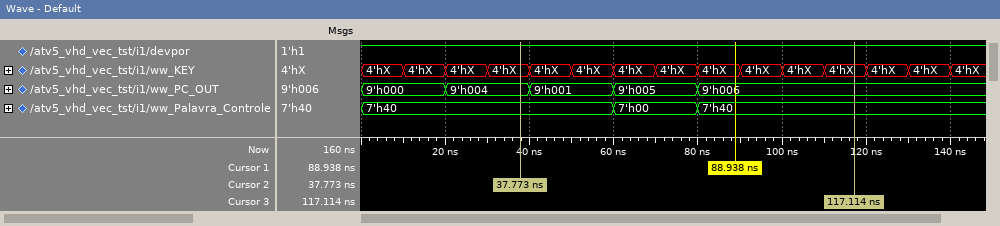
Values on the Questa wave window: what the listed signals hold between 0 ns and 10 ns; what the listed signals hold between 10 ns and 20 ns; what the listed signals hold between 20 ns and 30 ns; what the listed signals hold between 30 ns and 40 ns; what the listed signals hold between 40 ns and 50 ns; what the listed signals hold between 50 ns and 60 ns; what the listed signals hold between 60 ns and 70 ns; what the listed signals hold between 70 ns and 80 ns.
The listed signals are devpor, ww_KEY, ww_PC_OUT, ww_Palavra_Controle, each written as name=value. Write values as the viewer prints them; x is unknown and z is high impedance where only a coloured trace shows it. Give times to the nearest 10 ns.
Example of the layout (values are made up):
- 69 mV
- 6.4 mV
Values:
- devpor=1, ww_KEY=4'hX, ww_PC_OUT=9'h000, ww_Palavra_Controle=7'h40
- devpor=1, ww_KEY=4'hX, ww_PC_OUT=9'h000, ww_Palavra_Controle=7'h40
- devpor=1, ww_KEY=4'hX, ww_PC_OUT=9'h004, ww_Palavra_Controle=7'h40
- devpor=1, ww_KEY=4'hX, ww_PC_OUT=9'h004, ww_Palavra_Controle=7'h40
- devpor=1, ww_KEY=4'hX, ww_PC_OUT=9'h001, ww_Palavra_Controle=7'h40
- devpor=1, ww_KEY=4'hX, ww_PC_OUT=9'h001, ww_Palavra_Controle=7'h40
- devpor=1, ww_KEY=4'hX, ww_PC_OUT=9'h005, ww_Palavra_Controle=7'h00
- devpor=1, ww_KEY=4'hX, ww_PC_OUT=9'h005, ww_Palavra_Controle=7'h00
